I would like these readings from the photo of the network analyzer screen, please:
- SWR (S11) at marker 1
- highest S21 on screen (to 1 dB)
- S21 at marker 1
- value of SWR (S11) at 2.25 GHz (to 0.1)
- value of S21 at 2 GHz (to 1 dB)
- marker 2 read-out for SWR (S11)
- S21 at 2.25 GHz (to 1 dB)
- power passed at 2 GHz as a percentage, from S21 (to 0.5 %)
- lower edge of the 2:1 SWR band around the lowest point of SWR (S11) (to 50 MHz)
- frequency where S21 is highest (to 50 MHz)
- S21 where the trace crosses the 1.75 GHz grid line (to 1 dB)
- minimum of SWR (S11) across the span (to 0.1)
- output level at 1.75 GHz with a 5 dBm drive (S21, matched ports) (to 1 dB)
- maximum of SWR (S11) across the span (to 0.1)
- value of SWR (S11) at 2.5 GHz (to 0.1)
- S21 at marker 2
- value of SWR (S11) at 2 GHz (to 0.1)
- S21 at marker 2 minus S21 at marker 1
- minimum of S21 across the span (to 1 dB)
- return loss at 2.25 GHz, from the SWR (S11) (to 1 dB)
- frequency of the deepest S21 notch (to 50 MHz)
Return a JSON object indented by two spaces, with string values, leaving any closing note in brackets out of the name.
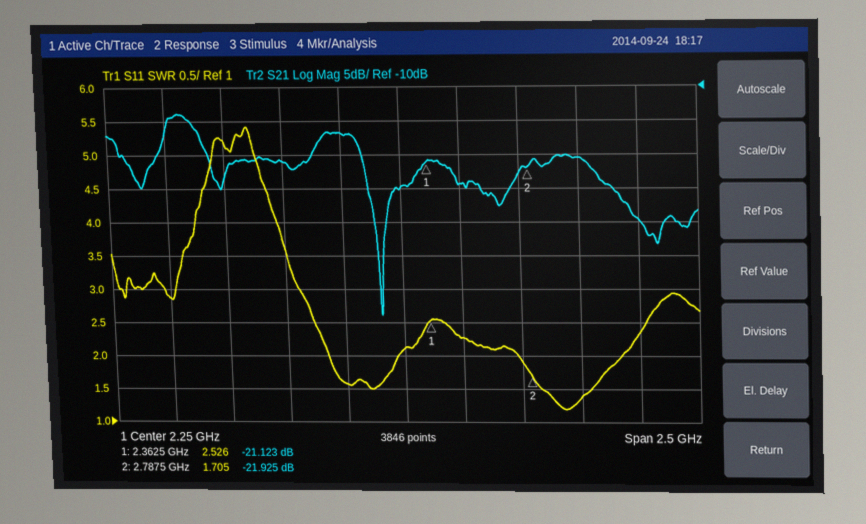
{
  "SWR (S11) at marker 1": "2.526",
  "highest S21 on screen": "-14 dB",
  "S21 at marker 1": "-21.123 dB",
  "value of SWR (S11) at 2.25 GHz": "2.1",
  "value of S21 at 2 GHz": "-17 dB",
  "marker 2 read-out for SWR": "1.705",
  "S21 at 2.25 GHz": "-25 dB",
  "power passed at 2 GHz as a percentage, from S21": "2.0 %",
  "lower edge of the 2:1 SWR band around the lowest point of SWR (S11)": "2.75 GHz",
  "frequency where S21 is highest": "1.30 GHz",
  "S21 where the trace crosses the 1.75 GHz grid line": "-21 dB",
  "minimum of SWR (S11) across the span": "1.2",
  "output level at 1.75 GHz with a 5 dBm drive (S21, matched ports)": "-16 dBm",
  "maximum of SWR (S11) across the span": "5.4",
  "value of SWR (S11) at 2.5 GHz": "2.3",
  "S21 at marker 2": "-21.925 dB",
  "value of SWR (S11) at 2 GHz": "1.6",
  "S21 at marker 2 minus S21 at marker 1": "-0.802 dB",
  "minimum of S21 across the span": "-44 dB",
  "return loss at 2.25 GHz, from the SWR (S11)": "9 dB",
  "frequency of the deepest S21 notch": "2.15 GHz"
}
